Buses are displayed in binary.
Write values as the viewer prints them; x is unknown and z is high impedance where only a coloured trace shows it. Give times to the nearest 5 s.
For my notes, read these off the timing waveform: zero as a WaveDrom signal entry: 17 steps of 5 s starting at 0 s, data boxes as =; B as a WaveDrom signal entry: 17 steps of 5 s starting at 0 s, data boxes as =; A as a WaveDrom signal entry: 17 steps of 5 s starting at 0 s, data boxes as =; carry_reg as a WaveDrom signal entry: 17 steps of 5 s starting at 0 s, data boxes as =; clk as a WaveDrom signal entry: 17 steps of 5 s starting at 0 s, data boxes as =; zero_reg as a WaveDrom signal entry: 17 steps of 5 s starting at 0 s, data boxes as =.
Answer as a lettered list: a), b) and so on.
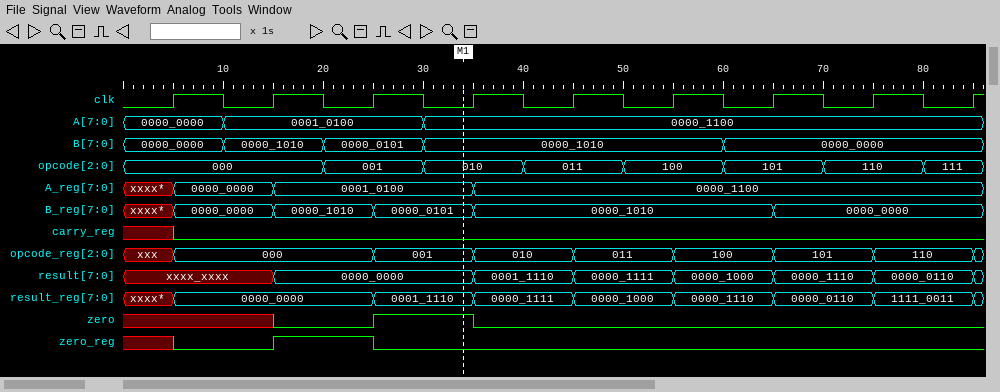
a) {name: 'zero', wave: 'x..0.1.0.........'}
b) {name: 'B', wave: '=.=.=.=.....=....', data: '0000_0000 0000_1010 0000_0101 0000_1010 0000_0000'}
c) {name: 'A', wave: '=.=...=..........', data: '0000_0000 0001_0100 0000_1100'}
d) {name: 'carry_reg', wave: 'x0...............'}
e) {name: 'clk', wave: '01010101010101010'}
f) {name: 'zero_reg', wave: 'x0.1.0...........'}
